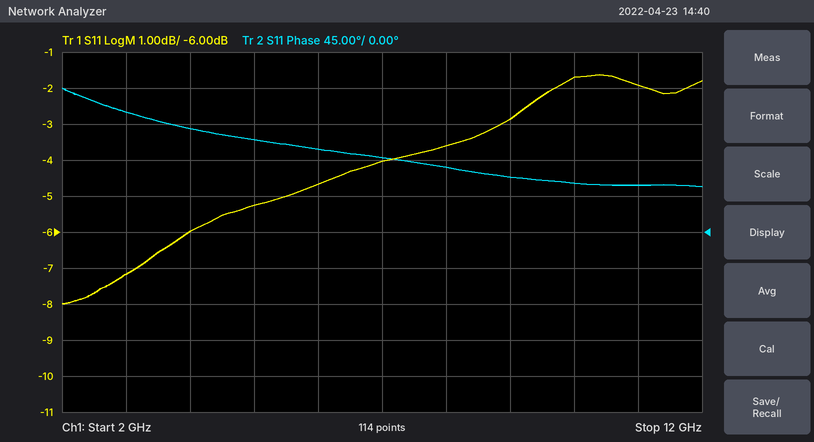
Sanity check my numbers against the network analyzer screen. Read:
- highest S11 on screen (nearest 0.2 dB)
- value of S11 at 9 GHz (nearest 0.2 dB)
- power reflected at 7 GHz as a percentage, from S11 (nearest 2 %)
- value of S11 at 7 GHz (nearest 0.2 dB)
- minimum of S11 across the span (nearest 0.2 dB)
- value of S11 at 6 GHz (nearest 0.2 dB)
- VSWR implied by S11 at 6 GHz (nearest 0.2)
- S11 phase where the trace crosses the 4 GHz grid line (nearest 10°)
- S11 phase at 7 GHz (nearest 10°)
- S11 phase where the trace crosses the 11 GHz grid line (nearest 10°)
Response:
-1.6 dB
-2.8 dB
40 %
-4.0 dB
-8.0 dB
-4.6 dB
3.8
130°
90°
60°
